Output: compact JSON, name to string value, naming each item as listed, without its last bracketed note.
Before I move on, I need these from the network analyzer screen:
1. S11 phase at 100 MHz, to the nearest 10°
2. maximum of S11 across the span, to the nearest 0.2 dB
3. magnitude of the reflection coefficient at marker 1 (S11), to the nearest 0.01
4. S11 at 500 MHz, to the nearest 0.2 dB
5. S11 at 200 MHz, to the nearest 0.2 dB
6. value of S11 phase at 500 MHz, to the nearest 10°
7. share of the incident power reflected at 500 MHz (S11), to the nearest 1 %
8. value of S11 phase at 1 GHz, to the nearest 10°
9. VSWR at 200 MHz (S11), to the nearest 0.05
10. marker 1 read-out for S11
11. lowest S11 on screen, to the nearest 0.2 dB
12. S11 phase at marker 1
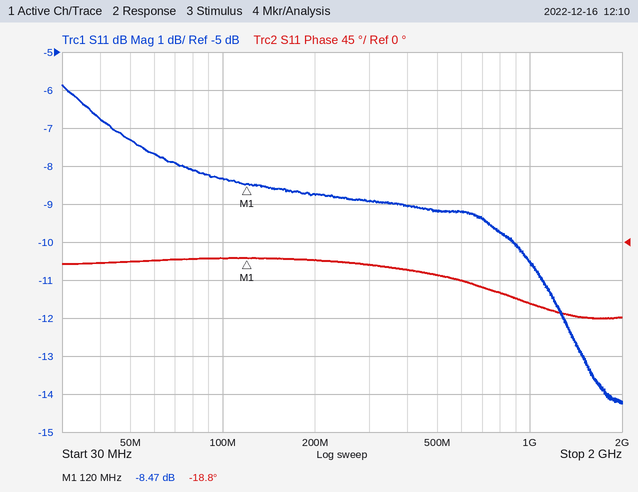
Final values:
{"S11 phase at 100 MHz, to the nearest 10°": "-20°", "maximum of S11 across the span, to the nearest 0.2 dB": "-5.8 dB", "magnitude of the reflection coefficient at marker 1 (S11), to the nearest 0.01": "0.38", "S11 at 500 MHz, to the nearest 0.2 dB": "-9.2 dB", "S11 at 200 MHz, to the nearest 0.2 dB": "-8.8 dB", "value of S11 phase at 500 MHz, to the nearest 10°": "-40°", "share of the incident power reflected at 500 MHz (S11), to the nearest 1 %": "12 %", "value of S11 phase at 1 GHz, to the nearest 10°": "-70°", "VSWR at 200 MHz (S11), to the nearest 0.05": "2.15", "marker 1 read-out for S11": "-8.47 dB", "lowest S11 on screen, to the nearest 0.2 dB": "-14.2 dB", "S11 phase at marker 1": "-18.8°"}
